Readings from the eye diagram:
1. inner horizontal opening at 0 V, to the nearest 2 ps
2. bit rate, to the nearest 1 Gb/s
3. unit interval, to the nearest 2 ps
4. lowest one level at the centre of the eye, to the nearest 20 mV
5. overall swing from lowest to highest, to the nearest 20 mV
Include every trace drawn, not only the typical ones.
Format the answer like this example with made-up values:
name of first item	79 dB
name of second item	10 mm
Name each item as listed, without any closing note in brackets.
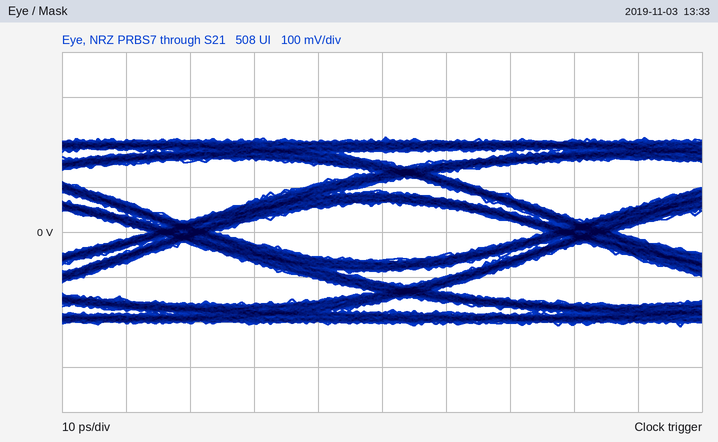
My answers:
inner horizontal opening at 0 V, to the nearest 2 ps	52 ps
bit rate, to the nearest 1 Gb/s	16 Gb/s
unit interval, to the nearest 2 ps	62 ps
lowest one level at the centre of the eye, to the nearest 20 mV	60 mV
overall swing from lowest to highest, to the nearest 20 mV	420 mV
